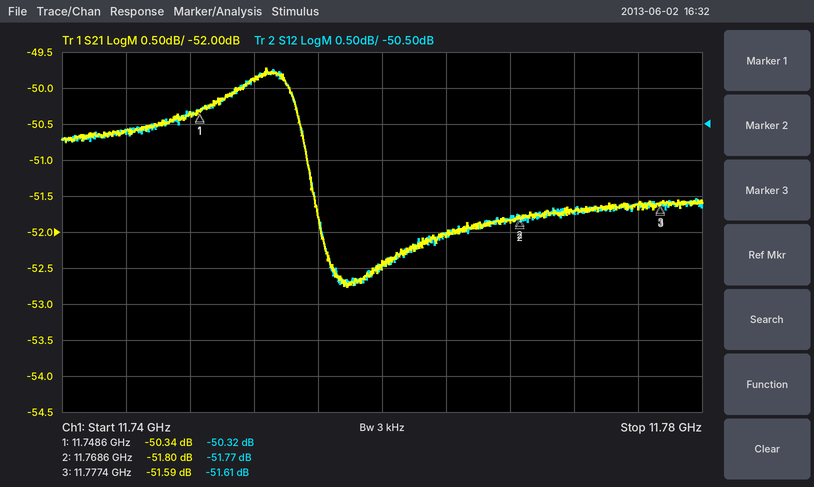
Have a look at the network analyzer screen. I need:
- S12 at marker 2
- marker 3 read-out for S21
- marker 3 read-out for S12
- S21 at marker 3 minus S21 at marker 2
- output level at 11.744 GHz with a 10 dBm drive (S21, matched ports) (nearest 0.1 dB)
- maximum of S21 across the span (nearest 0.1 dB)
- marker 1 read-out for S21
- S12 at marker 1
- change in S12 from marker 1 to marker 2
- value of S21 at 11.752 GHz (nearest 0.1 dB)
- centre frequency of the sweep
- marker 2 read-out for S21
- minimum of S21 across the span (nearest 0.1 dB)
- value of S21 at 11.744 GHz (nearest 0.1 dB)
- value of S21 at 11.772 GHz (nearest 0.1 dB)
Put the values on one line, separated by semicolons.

-51.77 dB; -51.59 dB; -51.61 dB; 0.21 dB; -40.6 dBm; -49.7 dB; -50.34 dB; -50.32 dB; -1.45 dB; -49.9 dB; 11.76 GHz; -51.80 dB; -52.8 dB; -50.6 dB; -51.7 dB
